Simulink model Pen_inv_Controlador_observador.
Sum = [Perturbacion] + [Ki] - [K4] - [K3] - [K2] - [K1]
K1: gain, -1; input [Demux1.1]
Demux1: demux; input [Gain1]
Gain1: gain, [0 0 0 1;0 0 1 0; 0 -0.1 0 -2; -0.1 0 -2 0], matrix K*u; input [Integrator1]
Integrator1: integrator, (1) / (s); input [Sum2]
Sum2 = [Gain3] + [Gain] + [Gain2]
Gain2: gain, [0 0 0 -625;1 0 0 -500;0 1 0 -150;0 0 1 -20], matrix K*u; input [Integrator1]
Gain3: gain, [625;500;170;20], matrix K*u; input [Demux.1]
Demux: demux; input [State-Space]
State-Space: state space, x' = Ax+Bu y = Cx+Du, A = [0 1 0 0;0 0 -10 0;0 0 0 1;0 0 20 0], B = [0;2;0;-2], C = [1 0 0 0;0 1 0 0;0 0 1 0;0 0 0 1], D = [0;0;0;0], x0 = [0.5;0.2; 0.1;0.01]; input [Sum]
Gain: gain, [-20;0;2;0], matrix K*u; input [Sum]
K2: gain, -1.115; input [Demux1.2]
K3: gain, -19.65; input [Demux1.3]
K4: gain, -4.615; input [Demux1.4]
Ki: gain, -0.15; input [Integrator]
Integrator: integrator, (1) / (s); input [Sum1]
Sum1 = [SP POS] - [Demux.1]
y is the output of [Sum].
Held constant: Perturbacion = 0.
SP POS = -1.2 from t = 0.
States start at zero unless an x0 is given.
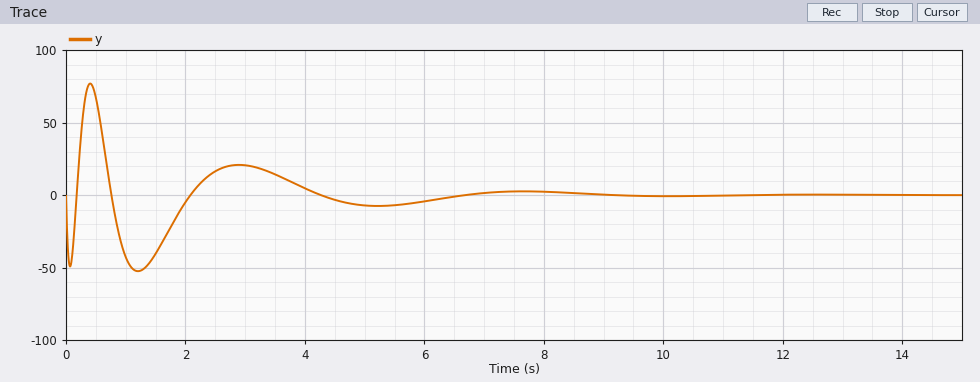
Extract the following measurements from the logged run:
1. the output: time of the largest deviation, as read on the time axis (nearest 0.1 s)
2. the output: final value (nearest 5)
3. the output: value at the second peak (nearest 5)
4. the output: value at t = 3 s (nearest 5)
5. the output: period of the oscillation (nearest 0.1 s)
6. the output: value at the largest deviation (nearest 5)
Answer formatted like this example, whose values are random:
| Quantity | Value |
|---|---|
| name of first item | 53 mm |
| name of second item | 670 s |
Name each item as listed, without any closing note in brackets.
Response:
| Quantity | Value |
|---|---|
| the output: time of the largest deviation, as read on the time axis | 0.4 s |
| the output: final value | 0 |
| the output: value at the second peak | 20 |
| the output: value at t = 3 s | 20 |
| the output: period of the oscillation | 2.5 s |
| the output: value at the largest deviation | 75 |
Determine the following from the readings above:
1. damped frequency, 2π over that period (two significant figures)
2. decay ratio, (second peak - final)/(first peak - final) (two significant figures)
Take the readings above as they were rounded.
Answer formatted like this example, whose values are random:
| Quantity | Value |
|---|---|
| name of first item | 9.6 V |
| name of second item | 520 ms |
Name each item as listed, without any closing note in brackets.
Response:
| Quantity | Value |
|---|---|
| damped frequency, 2π over that period | 2.5 rad/s |
| decay ratio, (second peak - final)/(first peak - final) | 0.27 |
